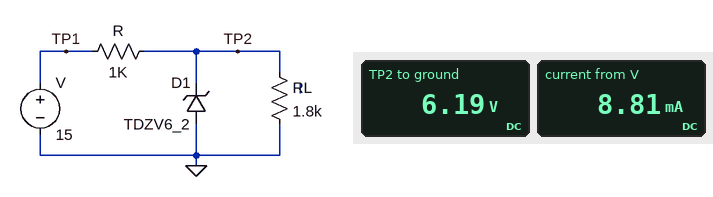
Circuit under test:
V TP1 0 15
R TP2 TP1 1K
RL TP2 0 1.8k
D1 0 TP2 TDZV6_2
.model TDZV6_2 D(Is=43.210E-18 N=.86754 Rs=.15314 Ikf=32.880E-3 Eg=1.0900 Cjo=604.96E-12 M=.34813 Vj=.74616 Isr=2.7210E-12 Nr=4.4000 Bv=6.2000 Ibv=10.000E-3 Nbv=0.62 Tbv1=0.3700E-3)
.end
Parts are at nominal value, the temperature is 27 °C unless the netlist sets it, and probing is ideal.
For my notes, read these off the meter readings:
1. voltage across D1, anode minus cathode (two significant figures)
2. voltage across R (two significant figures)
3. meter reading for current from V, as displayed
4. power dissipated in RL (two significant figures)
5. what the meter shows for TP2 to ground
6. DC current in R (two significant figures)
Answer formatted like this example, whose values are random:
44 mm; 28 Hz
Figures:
-6.2 V; 8.8 V; 8.81 mA; 21 mW; 6.19 V; 8.8 mA
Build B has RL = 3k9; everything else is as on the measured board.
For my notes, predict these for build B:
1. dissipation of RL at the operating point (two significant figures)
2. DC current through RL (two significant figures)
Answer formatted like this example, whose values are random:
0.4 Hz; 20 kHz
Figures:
9.8 mW; 1.6 mA
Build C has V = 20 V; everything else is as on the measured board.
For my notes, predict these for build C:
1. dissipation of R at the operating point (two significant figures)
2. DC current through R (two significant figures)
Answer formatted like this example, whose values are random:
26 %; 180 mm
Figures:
190 mW; 14 mA
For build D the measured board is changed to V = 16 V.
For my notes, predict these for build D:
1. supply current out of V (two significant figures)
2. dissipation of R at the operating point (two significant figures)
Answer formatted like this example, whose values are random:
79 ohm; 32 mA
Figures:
9.8 mA; 96 mW
